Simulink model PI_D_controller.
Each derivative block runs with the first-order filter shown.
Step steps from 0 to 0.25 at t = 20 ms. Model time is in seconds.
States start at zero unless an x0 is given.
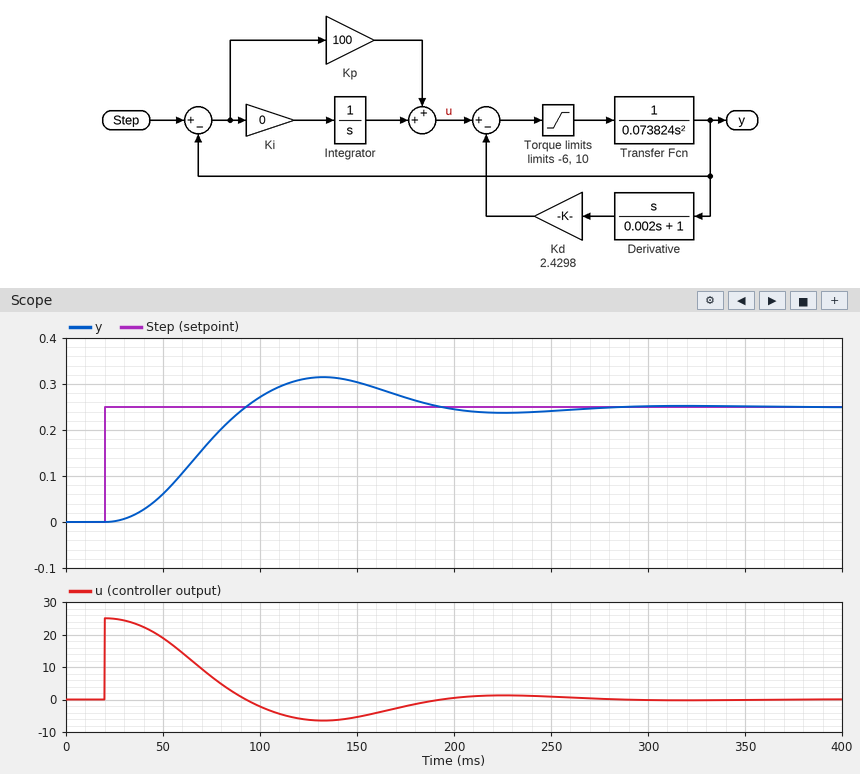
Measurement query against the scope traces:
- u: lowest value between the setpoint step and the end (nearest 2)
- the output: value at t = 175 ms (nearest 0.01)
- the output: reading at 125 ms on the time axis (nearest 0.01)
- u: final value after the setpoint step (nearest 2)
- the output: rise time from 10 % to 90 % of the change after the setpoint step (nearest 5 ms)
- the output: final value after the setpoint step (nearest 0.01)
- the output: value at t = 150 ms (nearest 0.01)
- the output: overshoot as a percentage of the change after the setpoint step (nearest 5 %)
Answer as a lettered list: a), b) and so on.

a) -6
b) 0.27
c) 0.31
d) 0
e) 45 ms
f) 0.25
g) 0.30
h) 25 %
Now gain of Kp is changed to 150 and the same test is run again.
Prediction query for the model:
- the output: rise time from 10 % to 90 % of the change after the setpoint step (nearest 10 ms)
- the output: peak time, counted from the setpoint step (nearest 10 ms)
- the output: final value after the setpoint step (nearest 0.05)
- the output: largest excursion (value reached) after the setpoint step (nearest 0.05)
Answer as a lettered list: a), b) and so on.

a) 40 ms
b) 120 ms
c) 0.25
d) 0.40
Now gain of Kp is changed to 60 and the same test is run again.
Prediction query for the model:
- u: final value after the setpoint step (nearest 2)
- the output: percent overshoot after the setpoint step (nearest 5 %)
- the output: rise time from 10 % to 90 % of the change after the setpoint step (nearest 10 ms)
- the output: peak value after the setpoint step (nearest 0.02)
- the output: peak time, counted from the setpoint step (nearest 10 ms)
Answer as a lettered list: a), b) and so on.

a) 0
b) 10 %
c) 60 ms
d) 0.28
e) 140 ms
